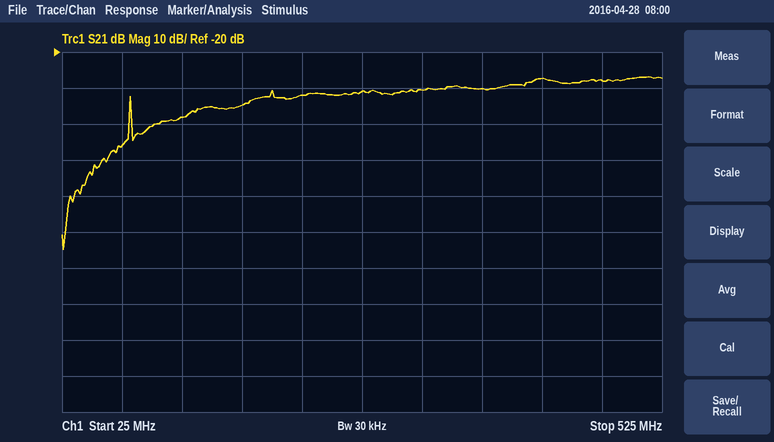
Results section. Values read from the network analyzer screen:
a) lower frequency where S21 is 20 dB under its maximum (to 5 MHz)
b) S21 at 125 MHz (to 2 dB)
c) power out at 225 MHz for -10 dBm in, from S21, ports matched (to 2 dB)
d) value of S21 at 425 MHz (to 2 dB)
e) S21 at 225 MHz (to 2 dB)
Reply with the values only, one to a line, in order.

70 MHz
-38 dB
-42 dBm
-28 dB
-32 dB
